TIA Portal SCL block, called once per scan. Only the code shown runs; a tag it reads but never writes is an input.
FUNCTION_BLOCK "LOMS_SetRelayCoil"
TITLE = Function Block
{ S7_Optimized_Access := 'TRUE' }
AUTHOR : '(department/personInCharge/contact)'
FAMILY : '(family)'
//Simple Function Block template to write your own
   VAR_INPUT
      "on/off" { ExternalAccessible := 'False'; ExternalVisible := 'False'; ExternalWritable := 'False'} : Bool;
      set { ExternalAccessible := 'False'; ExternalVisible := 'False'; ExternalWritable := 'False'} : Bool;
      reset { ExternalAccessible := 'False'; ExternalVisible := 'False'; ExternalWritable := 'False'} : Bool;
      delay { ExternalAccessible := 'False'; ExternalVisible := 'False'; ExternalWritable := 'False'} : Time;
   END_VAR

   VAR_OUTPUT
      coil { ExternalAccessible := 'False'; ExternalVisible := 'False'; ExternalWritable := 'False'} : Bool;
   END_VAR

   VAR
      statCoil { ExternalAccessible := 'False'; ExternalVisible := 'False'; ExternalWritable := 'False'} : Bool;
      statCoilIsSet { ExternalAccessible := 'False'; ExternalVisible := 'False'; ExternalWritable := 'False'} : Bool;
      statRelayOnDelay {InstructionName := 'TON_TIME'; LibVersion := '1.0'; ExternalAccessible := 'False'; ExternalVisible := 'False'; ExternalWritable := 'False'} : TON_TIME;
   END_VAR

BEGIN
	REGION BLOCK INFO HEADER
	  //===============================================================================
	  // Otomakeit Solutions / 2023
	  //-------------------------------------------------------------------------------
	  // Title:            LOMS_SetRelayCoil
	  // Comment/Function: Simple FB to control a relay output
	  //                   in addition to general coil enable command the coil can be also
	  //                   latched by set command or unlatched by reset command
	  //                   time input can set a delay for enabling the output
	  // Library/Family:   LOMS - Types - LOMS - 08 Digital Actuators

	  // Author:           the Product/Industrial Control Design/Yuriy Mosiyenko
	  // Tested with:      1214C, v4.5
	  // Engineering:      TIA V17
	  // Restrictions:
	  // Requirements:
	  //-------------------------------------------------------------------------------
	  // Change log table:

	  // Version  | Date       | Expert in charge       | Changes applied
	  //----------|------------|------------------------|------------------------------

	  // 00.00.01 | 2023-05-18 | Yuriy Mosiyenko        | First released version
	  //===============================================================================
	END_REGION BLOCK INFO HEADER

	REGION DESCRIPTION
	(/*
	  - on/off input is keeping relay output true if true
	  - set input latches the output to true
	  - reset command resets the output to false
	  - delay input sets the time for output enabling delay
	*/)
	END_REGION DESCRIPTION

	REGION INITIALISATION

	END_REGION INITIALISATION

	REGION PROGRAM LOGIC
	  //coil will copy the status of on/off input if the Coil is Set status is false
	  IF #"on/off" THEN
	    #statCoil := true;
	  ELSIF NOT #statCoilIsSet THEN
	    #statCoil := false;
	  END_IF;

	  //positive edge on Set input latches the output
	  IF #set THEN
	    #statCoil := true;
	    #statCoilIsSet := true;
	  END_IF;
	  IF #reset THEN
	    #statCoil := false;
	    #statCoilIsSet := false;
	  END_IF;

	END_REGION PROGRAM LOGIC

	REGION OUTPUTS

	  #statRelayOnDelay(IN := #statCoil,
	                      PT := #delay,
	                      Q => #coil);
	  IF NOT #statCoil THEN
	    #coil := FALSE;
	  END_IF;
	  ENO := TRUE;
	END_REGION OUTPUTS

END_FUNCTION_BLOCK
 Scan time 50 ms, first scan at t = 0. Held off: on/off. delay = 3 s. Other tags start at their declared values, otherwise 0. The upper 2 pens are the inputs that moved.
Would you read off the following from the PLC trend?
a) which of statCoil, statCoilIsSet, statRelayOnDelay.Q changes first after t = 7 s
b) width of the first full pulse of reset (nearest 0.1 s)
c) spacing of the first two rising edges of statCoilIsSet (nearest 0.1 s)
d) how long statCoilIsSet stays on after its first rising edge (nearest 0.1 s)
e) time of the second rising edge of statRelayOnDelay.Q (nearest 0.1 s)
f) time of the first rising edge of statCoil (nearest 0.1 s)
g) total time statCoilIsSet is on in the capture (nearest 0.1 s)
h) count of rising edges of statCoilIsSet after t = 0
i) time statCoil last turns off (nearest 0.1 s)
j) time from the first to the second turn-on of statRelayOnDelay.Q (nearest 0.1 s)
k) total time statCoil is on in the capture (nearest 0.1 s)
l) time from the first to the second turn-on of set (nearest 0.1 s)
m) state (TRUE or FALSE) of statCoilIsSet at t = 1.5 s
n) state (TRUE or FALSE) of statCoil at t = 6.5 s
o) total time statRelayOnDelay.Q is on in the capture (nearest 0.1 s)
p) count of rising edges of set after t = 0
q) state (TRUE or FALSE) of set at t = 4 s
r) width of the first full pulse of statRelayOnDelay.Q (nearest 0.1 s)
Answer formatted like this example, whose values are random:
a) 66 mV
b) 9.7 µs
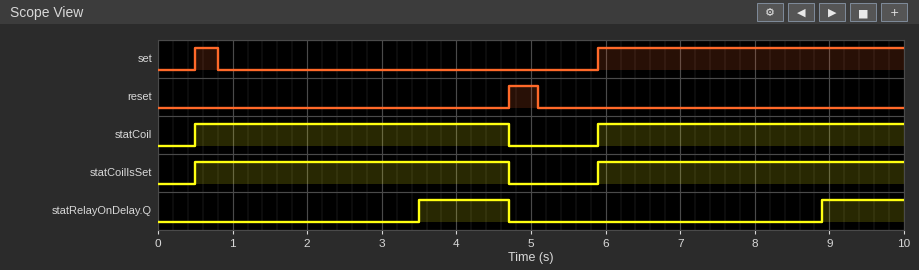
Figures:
a) statRelayOnDelay.Q
b) 0.4 s
c) 5.4 s
d) 4.2 s
e) 8.9 s
f) 0.5 s
g) 8.3 s
h) 2
i) 4.7 s
j) 5.4 s
k) 8.3 s
l) 5.4 s
m) TRUE
n) TRUE
o) 2.3 s
p) 2
q) FALSE
r) 1.2 s
